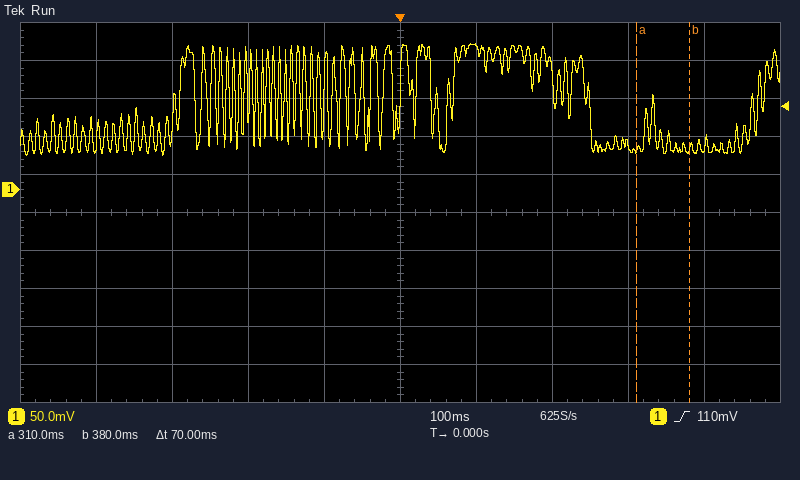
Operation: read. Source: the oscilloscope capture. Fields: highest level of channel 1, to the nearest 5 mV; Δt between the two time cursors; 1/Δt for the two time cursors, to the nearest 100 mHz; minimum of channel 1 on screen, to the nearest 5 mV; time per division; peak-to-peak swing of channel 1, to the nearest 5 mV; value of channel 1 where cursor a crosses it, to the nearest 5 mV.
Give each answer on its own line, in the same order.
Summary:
190 mV
70 ms
14.3 Hz
45 mV
100 ms
145 mV
55 mV
